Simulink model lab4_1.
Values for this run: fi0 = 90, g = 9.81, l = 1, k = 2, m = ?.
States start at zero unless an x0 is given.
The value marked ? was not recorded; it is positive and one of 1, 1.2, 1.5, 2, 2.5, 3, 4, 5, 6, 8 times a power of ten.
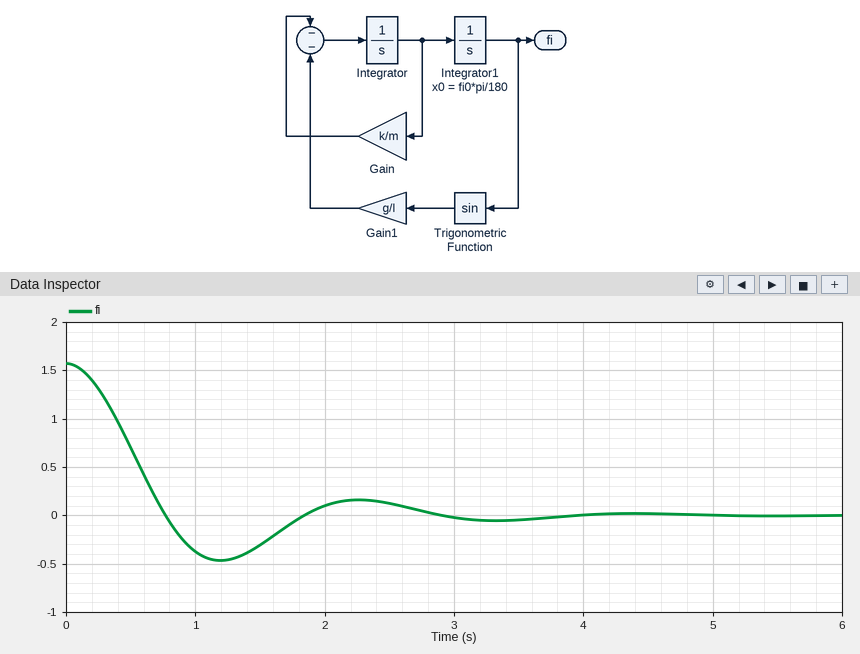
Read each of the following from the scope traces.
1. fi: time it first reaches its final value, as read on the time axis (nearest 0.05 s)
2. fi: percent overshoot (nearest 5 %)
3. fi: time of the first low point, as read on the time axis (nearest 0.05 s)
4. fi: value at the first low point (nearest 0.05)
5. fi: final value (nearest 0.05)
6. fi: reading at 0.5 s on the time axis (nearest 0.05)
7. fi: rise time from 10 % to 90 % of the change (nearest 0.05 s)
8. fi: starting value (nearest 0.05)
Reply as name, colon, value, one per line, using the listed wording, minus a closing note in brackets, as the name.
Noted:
fi: time it first reaches its final value, as read on the time axis: 0.75 s
fi: percent overshoot: 30 %
fi: time of the first low point, as read on the time axis: 1.20 s
fi: value at the first low point: -0.45
fi: final value: 0.00
fi: reading at 0.5 s on the time axis: 0.70
fi: rise time from 10 % to 90 % of the change: 0.50 s
fi: starting value: 1.55
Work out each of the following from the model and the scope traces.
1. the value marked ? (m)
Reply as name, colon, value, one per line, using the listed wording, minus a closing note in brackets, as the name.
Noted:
the value marked ?: 1
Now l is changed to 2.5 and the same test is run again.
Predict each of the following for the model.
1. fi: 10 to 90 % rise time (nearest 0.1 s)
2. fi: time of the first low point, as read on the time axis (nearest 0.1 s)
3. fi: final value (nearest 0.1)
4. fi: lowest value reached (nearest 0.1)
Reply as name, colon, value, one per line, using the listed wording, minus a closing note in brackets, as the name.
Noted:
fi: 10 to 90 % rise time: 1.0 s
fi: time of the first low point, as read on the time axis: 2.1 s
fi: final value: 0.0
fi: lowest value reached: -0.2
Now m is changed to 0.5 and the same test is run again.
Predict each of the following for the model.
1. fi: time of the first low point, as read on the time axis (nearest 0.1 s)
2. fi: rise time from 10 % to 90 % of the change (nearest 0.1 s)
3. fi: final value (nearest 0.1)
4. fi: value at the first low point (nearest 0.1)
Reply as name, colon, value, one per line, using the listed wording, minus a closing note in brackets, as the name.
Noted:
fi: time of the first low point, as read on the time axis: 1.5 s
fi: rise time from 10 % to 90 % of the change: 0.8 s
fi: final value: 0.0
fi: value at the first low point: -0.1
